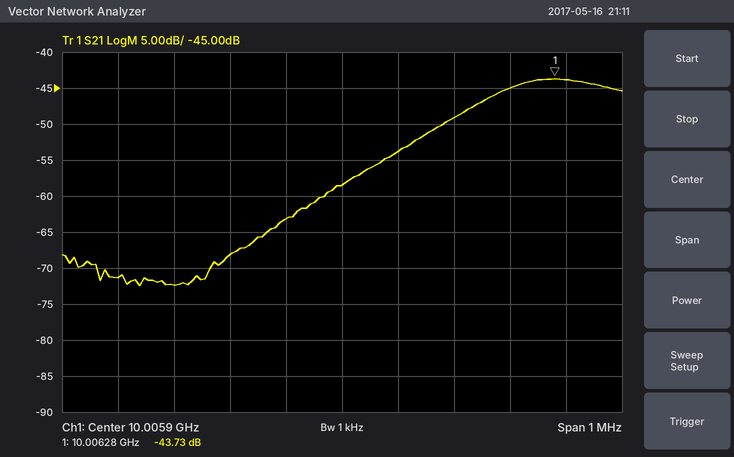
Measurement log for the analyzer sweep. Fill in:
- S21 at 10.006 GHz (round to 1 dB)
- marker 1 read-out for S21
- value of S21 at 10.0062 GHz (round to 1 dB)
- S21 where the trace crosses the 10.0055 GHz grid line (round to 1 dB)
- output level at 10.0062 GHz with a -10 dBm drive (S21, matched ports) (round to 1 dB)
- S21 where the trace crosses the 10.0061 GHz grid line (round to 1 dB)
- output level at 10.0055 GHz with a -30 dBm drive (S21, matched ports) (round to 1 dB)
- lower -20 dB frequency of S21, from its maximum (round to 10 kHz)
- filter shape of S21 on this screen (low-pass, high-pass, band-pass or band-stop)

-54 dB
-43.73 dB
-45 dB
-71 dB
-55 dBm
-49 dB
-101 dBm
10.00579 GHz
high-pass
